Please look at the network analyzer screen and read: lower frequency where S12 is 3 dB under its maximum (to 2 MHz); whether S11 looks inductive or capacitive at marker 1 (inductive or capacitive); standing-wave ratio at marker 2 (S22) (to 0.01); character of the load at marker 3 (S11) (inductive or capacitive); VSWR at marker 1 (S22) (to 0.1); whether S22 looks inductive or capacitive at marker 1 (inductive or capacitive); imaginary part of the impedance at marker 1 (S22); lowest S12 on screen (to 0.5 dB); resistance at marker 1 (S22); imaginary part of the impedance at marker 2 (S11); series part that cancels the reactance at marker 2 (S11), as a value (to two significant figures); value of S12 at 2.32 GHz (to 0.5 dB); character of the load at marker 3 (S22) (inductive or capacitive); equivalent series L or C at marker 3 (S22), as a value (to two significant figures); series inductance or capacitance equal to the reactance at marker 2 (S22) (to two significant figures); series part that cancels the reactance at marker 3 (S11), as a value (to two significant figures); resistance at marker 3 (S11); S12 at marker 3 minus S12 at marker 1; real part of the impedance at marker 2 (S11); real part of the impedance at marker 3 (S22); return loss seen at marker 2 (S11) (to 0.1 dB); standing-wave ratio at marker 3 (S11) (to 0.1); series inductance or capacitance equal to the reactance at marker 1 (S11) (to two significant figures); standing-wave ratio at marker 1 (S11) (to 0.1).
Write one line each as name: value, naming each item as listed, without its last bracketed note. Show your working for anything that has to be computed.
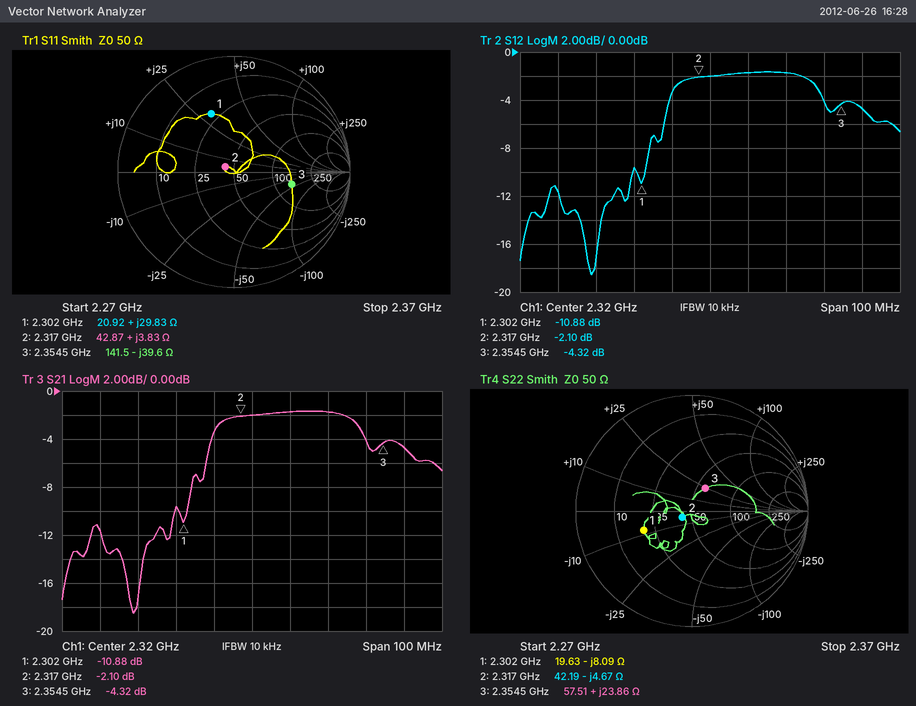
lower frequency where S12 is 3 dB under its maximum: 2.308 GHz
whether S11 looks inductive or capacitive at marker 1: inductive
standing-wave ratio at marker 2 (S22): 1.22
character of the load at marker 3 (S11): capacitive
VSWR at marker 1 (S22): 2.6
whether S22 looks inductive or capacitive at marker 1: capacitive
imaginary part of the impedance at marker 1: -8.09 Ω
lowest S12 on screen: -18.5 dB
resistance at marker 1: 19.63 Ω
imaginary part of the impedance at marker 2: +3.83 Ω
series part that cancels the reactance at marker 2 (S11), as a value: C = 1/(2π × 2.317 GHz × 3.83 Ω) ≈ 18 pF
value of S12 at 2.32 GHz: -2.0 dB
character of the load at marker 3 (S22): inductive
equivalent series L or C at marker 3 (S22), as a value: L = 23.86 Ω/(2π × 2.3545 GHz) ≈ 1.6 nH
series inductance or capacitance equal to the reactance at marker 2 (S22): C = 1/(2π × 2.317 GHz × 4.67 Ω) ≈ 15 pF
series part that cancels the reactance at marker 3 (S11), as a value: L = 39.6 Ω/(2π × 2.3545 GHz) ≈ 2.7 nH
resistance at marker 3: 141.5 Ω
S12 at marker 3 minus S12 at marker 1: -4.32 − (-10.88) = 6.56 dB
real part of the impedance at marker 2: 42.87 Ω
real part of the impedance at marker 3: 57.51 Ω
return loss seen at marker 2 (S11): 21.2 dB
standing-wave ratio at marker 3 (S11): 3.1
series inductance or capacitance equal to the reactance at marker 1 (S11): L = 29.83 Ω/(2π × 2.302 GHz) ≈ 2.1 nH
standing-wave ratio at marker 1 (S11): 3.4
